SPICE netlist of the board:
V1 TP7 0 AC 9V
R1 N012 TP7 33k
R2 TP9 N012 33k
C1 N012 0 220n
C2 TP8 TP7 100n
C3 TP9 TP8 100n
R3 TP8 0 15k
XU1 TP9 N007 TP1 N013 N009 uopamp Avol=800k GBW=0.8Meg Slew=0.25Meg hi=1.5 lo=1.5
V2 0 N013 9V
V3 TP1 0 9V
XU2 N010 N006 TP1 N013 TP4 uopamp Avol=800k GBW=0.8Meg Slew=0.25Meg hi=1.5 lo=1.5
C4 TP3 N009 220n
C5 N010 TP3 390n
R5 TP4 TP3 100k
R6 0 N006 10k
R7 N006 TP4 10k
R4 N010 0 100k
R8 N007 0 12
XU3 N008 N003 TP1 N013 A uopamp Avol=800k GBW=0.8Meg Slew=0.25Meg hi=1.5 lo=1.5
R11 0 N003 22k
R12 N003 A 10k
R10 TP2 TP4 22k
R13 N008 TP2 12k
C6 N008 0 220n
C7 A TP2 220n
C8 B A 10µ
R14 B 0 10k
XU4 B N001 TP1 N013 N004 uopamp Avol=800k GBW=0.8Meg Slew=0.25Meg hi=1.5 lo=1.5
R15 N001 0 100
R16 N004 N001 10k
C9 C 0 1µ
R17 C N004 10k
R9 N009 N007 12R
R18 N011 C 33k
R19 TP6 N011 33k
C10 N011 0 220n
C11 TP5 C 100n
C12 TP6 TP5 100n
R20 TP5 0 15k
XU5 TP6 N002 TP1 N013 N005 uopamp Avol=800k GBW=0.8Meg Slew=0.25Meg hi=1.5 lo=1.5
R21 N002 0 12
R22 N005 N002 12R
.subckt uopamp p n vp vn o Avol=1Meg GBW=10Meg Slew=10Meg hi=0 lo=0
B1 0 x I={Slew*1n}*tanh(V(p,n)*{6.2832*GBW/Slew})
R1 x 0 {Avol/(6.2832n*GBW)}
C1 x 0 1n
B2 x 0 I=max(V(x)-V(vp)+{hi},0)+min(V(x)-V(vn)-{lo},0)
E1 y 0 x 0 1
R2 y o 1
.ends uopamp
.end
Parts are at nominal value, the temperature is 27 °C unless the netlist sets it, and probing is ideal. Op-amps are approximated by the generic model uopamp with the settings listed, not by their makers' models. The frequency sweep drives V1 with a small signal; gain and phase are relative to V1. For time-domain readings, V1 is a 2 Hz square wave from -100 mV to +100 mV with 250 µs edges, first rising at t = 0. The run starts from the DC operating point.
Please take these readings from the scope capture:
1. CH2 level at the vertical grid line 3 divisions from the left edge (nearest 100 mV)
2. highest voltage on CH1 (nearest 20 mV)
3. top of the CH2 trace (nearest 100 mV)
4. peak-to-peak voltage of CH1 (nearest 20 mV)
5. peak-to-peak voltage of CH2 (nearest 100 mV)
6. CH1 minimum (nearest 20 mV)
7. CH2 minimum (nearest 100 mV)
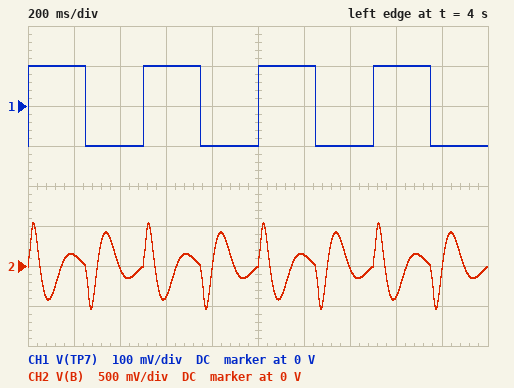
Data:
-400 mV
100 mV
500 mV
200 mV
1.1 V
-100 mV
-500 mV
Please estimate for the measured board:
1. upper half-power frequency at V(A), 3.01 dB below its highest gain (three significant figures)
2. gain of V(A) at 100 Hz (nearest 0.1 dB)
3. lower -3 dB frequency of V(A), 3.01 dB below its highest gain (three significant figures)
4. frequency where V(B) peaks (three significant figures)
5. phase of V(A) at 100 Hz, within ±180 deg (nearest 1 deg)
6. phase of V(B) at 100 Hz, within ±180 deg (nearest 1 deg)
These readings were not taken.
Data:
10.3 Hz
-7.9 dB
4.44 Hz
6.18 Hz
-66 deg
-65 deg
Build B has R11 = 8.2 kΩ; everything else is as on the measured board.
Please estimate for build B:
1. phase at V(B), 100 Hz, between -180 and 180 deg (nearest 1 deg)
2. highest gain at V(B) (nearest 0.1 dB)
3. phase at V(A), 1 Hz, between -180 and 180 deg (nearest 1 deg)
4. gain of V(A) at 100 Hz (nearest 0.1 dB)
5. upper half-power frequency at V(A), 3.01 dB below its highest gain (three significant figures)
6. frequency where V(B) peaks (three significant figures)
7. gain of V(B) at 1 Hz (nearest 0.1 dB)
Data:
-91 deg
20.9 dB
166 deg
-2.2 dB
10.8 Hz
6.23 Hz
-15.7 dB
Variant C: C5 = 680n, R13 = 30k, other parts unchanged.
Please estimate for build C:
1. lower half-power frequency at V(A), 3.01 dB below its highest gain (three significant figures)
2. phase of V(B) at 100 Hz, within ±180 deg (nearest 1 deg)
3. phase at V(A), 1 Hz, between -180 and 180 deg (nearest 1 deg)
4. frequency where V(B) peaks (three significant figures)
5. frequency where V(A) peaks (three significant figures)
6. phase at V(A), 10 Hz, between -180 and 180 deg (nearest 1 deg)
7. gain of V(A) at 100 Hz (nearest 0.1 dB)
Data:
3.46 Hz
-79 deg
163 deg
4.48 Hz
4.43 Hz
-61 deg
-15.8 dB
